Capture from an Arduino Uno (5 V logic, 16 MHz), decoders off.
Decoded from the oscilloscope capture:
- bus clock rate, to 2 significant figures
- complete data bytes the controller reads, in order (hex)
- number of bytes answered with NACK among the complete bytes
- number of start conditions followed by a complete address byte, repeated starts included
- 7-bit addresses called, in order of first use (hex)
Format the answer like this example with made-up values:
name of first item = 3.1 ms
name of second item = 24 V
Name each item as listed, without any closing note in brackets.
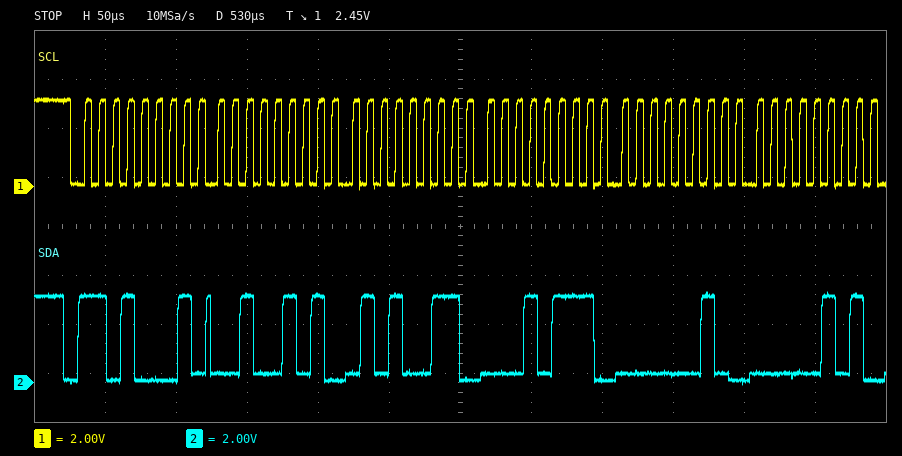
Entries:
bus clock rate, to 2 significant figures = 100 kHz
complete data bytes the controller reads, in order = 25 53 17 02 05
number of bytes answered with NACK among the complete bytes = 0
number of start conditions followed by a complete address byte, repeated starts included = 1
7-bit addresses called, in order of first use = 0x68
